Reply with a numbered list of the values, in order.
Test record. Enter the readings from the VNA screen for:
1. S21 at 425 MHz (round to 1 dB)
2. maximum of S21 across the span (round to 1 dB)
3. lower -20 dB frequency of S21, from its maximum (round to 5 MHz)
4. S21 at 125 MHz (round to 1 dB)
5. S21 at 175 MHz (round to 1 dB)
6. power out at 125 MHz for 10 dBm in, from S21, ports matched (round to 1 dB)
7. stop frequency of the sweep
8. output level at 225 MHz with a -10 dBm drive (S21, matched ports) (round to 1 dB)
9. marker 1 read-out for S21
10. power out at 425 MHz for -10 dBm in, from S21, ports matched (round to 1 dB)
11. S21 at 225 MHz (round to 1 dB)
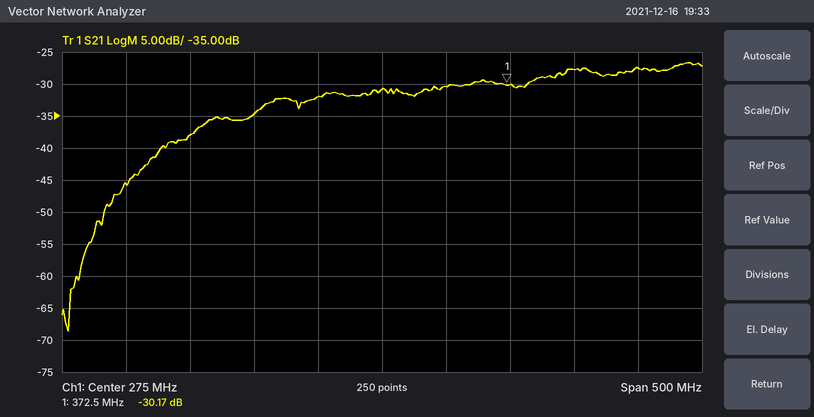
1. -28 dB
2. -27 dB
3. 70 MHz
4. -38 dB
5. -35 dB
6. -28 dBm
7. 525 MHz
8. -42 dBm
9. -30.17 dB
10. -38 dBm
11. -32 dB
